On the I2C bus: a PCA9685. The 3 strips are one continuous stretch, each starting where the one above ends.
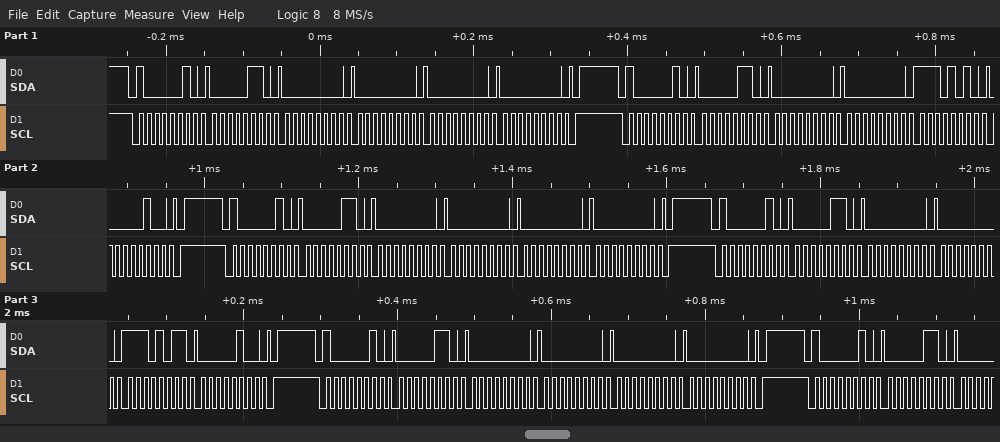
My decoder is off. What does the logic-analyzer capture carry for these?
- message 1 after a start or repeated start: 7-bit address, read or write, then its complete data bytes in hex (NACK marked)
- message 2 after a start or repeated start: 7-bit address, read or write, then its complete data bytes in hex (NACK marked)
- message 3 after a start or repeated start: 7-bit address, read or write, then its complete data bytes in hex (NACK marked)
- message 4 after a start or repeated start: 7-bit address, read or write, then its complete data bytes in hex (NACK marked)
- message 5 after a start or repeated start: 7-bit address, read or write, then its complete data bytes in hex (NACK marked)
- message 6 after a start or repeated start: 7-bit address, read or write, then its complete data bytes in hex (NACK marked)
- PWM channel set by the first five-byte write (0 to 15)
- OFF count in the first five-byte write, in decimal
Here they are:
0x41 write: 06 00 00 00 00
0x41 write: 06 00 00 EA 04
0x41 write: 06 00 00 00 00
0x41 write: 06 00 00 EB 04
0x41 write: 06 00 00 00 00
0x41 write: 06
0
0
